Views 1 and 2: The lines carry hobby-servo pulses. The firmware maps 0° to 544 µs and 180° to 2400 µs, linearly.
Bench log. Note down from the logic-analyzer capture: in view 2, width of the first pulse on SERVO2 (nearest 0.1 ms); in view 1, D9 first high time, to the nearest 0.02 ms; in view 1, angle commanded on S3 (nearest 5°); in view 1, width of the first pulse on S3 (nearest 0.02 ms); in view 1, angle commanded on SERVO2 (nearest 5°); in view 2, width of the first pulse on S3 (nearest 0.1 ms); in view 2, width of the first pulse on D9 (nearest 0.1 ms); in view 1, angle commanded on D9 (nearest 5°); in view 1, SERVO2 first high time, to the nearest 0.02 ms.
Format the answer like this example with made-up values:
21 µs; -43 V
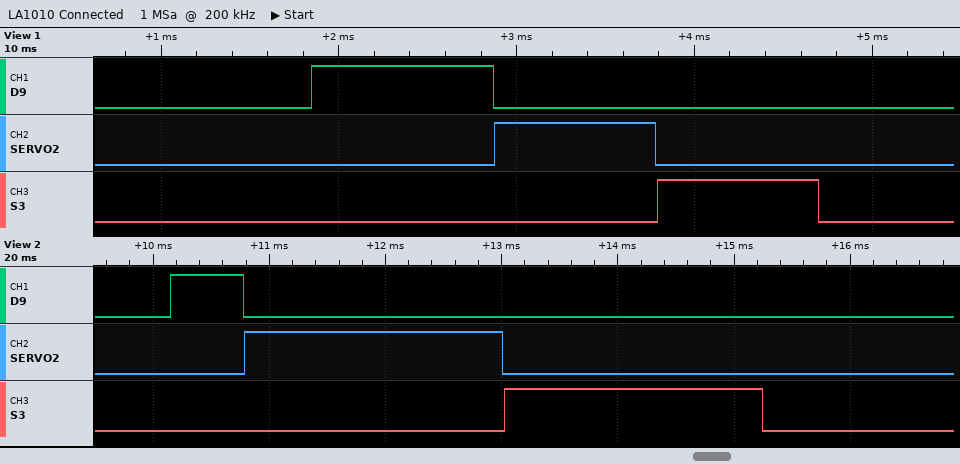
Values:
2.2 ms; 1.02 ms; 35°; 0.90 ms; 35°; 2.2 ms; 0.6 ms; 45°; 0.90 ms
